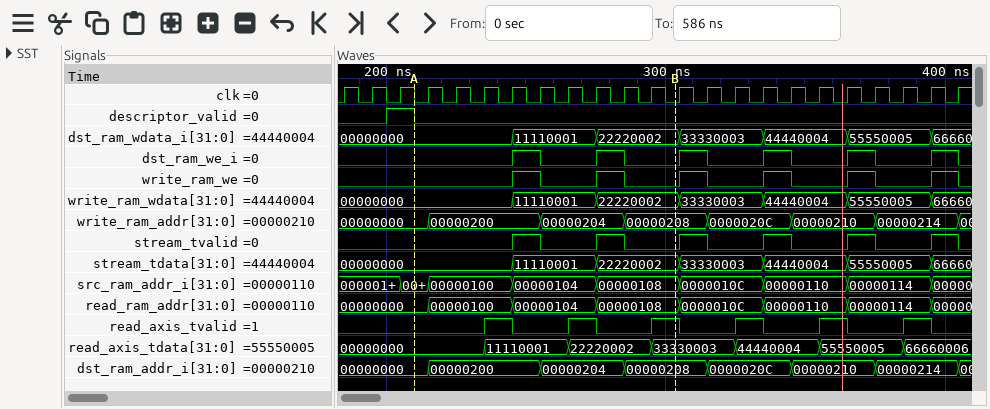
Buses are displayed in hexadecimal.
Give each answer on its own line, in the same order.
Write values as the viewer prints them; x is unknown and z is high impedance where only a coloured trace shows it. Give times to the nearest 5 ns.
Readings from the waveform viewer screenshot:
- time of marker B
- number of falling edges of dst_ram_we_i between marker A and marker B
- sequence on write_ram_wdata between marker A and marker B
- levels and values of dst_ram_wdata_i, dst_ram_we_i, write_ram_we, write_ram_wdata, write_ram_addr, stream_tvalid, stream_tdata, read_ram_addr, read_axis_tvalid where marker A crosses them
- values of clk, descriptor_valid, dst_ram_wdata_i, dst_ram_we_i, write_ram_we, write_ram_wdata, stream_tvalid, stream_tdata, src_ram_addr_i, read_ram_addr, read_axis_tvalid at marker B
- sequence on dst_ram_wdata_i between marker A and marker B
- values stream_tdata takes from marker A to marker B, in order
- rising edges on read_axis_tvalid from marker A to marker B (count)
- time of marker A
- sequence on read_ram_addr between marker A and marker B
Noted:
305 ns
2
00000000, 11110001, 22220002
dst_ram_wdata_i=00000000, dst_ram_we_i=0, write_ram_we=0, write_ram_wdata=00000000, write_ram_addr=00000000, stream_tvalid=0, stream_tdata=00000000, read_ram_addr=00000000, read_axis_tvalid=0
clk=0, descriptor_valid=0, dst_ram_wdata_i=22220002, dst_ram_we_i=0, write_ram_we=0, write_ram_wdata=22220002, stream_tvalid=0, stream_tdata=22220002, src_ram_addr_i=00000108, read_ram_addr=00000108, read_axis_tvalid=1
00000000, 11110001, 22220002
00000000, 11110001, 22220002
3
210 ns
00000000, 00000100, 00000104, 00000108
